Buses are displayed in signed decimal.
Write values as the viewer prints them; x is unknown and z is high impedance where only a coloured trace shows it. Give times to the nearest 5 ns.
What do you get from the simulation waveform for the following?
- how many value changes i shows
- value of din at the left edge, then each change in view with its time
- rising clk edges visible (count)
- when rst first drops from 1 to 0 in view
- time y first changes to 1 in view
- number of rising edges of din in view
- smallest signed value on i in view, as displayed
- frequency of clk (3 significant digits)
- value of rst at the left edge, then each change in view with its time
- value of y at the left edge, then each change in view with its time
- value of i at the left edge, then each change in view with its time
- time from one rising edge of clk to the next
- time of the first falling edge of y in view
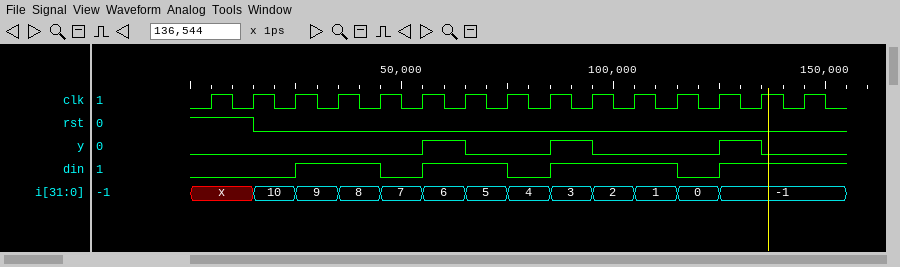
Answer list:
12
0, 1 at 25 ns, 0 at 45 ns, 1 at 55 ns, 0 at 75 ns, 1 at 85 ns, 0 at 115 ns, 1 at 125 ns
15
15 ns
55 ns
4
-1
100 MHz
1, 0 at 15 ns
0, 1 at 55 ns, 0 at 65 ns, 1 at 85 ns, 0 at 95 ns, 1 at 125 ns, 0 at 135 ns
x, 10 at 15 ns, 9 at 25 ns, 8 at 35 ns, 7 at 45 ns, 6 at 55 ns, 5 at 65 ns, 4 at 75 ns, 3 at 85 ns, 2 at 95 ns, 1 at 105 ns, 0 at 115 ns, -1 at 125 ns
10 ns
65 ns
